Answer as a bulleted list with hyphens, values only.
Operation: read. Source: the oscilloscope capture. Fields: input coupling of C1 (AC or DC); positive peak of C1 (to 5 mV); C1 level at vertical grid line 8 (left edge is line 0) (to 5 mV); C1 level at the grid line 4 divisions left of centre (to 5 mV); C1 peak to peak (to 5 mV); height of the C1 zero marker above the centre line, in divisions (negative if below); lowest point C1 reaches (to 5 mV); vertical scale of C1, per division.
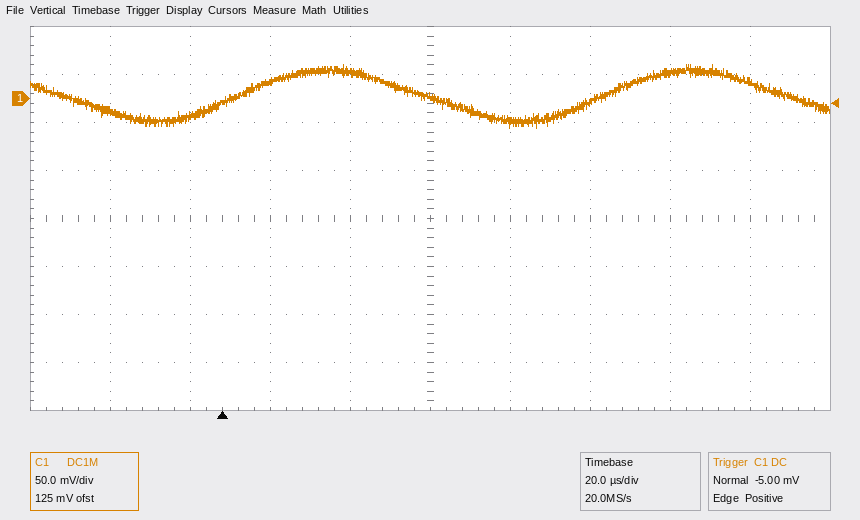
- DC
- 35 mV
- 25 mV
- -15 mV
- 65 mV
- +2.5 div
- -30 mV
- 50 mV
